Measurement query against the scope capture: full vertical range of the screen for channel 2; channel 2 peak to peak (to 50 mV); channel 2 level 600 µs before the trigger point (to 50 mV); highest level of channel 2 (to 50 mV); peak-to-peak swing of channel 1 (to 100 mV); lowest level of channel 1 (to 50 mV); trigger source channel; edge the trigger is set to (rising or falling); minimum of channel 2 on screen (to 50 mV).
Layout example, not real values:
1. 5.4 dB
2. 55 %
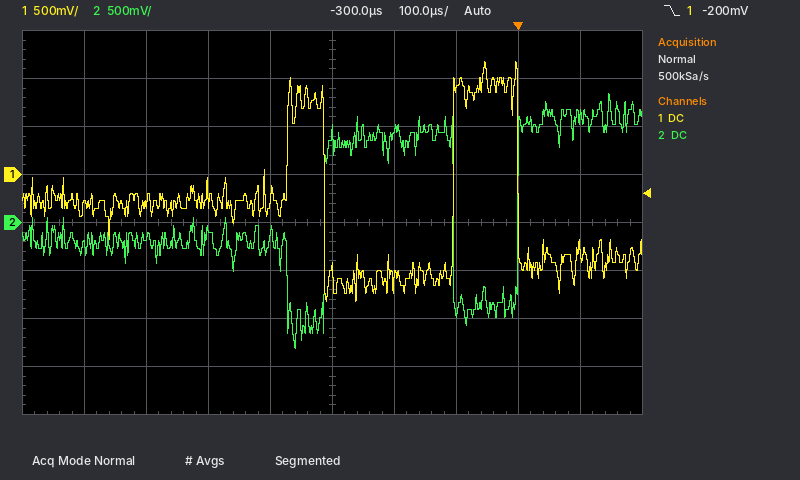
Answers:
1. 4 V
2. 2.65 V
3. -150 mV
4. 1.35 V
5. 2.50 V
6. -1.30 V
7. channel 1
8. falling
9. -1.30 V
